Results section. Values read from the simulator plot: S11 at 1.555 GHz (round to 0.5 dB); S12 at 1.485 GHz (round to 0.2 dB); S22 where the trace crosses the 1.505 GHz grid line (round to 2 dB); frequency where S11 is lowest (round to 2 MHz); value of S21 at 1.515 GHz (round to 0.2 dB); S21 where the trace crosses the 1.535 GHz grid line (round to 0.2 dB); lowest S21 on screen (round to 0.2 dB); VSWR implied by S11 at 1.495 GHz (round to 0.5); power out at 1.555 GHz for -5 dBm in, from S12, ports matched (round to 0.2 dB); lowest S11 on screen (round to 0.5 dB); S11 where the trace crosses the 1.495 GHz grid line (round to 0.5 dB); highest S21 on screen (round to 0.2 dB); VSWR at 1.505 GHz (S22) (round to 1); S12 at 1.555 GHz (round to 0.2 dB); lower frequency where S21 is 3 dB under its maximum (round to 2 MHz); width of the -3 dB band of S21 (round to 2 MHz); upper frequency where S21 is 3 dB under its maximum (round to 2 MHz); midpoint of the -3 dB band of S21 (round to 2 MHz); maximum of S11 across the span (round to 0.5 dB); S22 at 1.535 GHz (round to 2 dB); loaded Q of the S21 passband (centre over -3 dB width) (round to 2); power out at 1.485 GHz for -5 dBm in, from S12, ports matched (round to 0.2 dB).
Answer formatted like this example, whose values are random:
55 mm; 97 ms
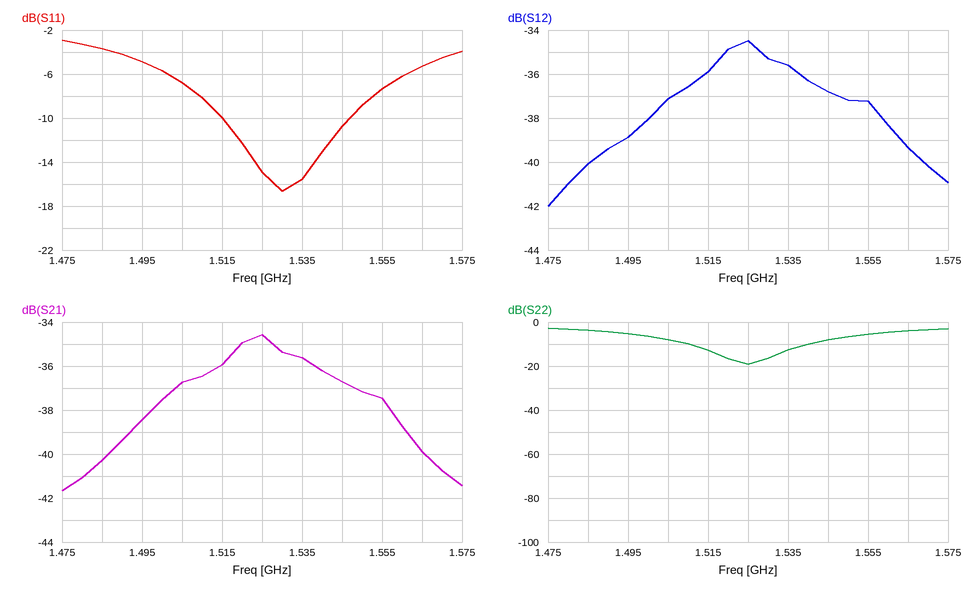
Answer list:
-7.5 dB; -40.0 dB; -8 dB; 1.530 GHz; -36.0 dB; -35.6 dB; -41.6 dB; 3.5; -42.2 dBm; -16.5 dB; -5.0 dB; -34.6 dB; 2; -37.2 dB; 1.500 GHz; 56 MHz; 1.556 GHz; 1.528 GHz; -3.0 dB; -12 dB; 28; -45.0 dBm
